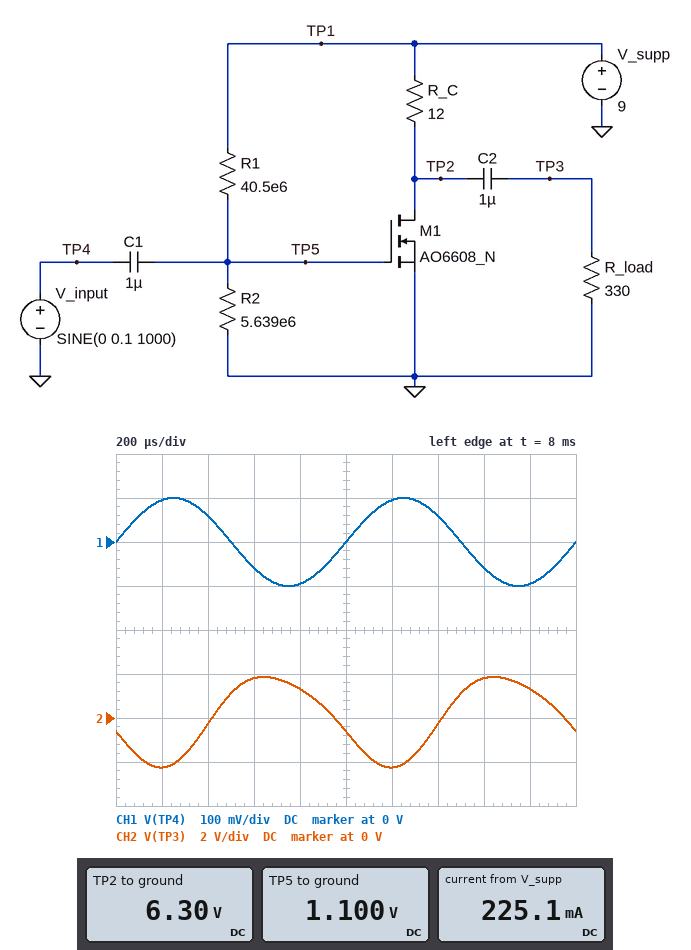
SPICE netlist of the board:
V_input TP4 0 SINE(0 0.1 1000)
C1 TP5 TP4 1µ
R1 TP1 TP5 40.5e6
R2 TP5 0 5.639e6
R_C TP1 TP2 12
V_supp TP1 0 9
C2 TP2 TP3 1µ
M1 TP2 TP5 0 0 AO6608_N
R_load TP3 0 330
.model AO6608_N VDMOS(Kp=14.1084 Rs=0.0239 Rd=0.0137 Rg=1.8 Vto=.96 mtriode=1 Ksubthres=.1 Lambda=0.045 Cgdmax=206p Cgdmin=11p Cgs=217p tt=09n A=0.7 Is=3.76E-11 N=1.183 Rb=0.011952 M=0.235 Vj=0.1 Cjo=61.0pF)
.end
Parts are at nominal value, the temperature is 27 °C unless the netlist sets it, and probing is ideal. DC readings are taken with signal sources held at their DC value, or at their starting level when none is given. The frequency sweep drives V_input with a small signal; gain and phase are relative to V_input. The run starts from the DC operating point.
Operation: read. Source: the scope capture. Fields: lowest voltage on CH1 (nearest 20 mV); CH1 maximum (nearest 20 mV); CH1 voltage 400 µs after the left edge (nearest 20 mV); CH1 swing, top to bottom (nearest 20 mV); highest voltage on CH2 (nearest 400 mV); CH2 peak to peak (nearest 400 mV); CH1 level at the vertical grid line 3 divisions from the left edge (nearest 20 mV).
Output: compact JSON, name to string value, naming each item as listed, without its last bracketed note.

{"lowest voltage on CH1": "-100 mV", "CH1 maximum": "100 mV", "CH1 voltage 400 µs after the left edge": "60 mV", "CH1 swing, top to bottom": "200 mV", "highest voltage on CH2": "2.0 V", "CH2 peak to peak": "4.0 V", "CH1 level at the vertical grid line 3 divisions from the left edge": "-60 mV"}
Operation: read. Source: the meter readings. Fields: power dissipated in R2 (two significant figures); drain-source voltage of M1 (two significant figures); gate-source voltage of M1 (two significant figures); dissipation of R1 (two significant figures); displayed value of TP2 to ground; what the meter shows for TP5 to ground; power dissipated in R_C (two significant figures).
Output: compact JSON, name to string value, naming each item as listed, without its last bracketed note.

{"power dissipated in R2": "210 nW", "drain-source voltage of M1": "6.3 V", "gate-source voltage of M1": "1.1 V", "dissipation of R1": "1.5 µW", "displayed value of TP2 to ground": "6.30 V", "what the meter shows for TP5 to ground": "1.100 V", "power dissipated in R_C": "610 mW"}
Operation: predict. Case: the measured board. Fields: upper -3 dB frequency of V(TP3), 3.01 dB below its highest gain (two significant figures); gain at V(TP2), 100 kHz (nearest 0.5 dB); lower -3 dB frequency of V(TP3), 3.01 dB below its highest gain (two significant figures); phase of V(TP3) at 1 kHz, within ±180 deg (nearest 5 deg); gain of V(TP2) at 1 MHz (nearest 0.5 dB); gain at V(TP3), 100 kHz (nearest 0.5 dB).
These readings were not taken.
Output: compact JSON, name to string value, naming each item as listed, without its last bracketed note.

{"upper -3 dB frequency of V(TP3), 3.01 dB below its highest gain": "72 MHz", "gain at V(TP2), 100 kHz": "27.0 dB", "lower -3 dB frequency of V(TP3), 3.01 dB below its highest gain": "470 Hz", "phase of V(TP3) at 1 kHz, within ±180 deg": "-155 deg", "gain of V(TP2) at 1 MHz": "27.0 dB", "gain at V(TP3), 100 kHz": "27.0 dB"}
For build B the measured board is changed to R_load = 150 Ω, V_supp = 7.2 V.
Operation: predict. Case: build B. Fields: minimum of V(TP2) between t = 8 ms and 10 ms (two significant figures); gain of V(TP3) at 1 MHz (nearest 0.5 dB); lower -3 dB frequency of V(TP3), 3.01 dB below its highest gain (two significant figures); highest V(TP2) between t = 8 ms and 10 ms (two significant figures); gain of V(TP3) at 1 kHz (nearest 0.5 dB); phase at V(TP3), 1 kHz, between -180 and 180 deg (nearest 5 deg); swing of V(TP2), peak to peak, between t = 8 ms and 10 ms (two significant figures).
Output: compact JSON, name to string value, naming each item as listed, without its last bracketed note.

{"minimum of V(TP2) between t = 8 ms and 10 ms": "6.5 V", "gain of V(TP3) at 1 MHz": "7.5 dB", "lower -3 dB frequency of V(TP3), 3.01 dB below its highest gain": "980 Hz", "highest V(TP2) between t = 8 ms and 10 ms": "7.2 V", "gain of V(TP3) at 1 kHz": "4.5 dB", "phase at V(TP3), 1 kHz, between -180 and 180 deg": "-135 deg", "swing of V(TP2), peak to peak, between t = 8 ms and 10 ms": "630 mV"}
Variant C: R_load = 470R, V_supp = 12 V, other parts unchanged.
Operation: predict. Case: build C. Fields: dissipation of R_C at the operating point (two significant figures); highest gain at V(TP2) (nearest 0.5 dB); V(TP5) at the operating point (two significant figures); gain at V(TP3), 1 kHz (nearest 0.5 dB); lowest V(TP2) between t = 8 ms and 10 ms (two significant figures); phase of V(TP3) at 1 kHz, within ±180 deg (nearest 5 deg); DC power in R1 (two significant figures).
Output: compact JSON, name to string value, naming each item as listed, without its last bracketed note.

{"dissipation of R_C at the operating point": "12 W", "highest gain at V(TP2)": "-5.5 dB", "V(TP5) at the operating point": "1.5 V", "gain at V(TP3), 1 kHz": "-6.0 dB", "lowest V(TP2) between t = 8 ms and 10 ms": "170 mV", "phase of V(TP3) at 1 kHz, within ±180 deg": "-160 deg", "DC power in R1": "2.7 µW"}
